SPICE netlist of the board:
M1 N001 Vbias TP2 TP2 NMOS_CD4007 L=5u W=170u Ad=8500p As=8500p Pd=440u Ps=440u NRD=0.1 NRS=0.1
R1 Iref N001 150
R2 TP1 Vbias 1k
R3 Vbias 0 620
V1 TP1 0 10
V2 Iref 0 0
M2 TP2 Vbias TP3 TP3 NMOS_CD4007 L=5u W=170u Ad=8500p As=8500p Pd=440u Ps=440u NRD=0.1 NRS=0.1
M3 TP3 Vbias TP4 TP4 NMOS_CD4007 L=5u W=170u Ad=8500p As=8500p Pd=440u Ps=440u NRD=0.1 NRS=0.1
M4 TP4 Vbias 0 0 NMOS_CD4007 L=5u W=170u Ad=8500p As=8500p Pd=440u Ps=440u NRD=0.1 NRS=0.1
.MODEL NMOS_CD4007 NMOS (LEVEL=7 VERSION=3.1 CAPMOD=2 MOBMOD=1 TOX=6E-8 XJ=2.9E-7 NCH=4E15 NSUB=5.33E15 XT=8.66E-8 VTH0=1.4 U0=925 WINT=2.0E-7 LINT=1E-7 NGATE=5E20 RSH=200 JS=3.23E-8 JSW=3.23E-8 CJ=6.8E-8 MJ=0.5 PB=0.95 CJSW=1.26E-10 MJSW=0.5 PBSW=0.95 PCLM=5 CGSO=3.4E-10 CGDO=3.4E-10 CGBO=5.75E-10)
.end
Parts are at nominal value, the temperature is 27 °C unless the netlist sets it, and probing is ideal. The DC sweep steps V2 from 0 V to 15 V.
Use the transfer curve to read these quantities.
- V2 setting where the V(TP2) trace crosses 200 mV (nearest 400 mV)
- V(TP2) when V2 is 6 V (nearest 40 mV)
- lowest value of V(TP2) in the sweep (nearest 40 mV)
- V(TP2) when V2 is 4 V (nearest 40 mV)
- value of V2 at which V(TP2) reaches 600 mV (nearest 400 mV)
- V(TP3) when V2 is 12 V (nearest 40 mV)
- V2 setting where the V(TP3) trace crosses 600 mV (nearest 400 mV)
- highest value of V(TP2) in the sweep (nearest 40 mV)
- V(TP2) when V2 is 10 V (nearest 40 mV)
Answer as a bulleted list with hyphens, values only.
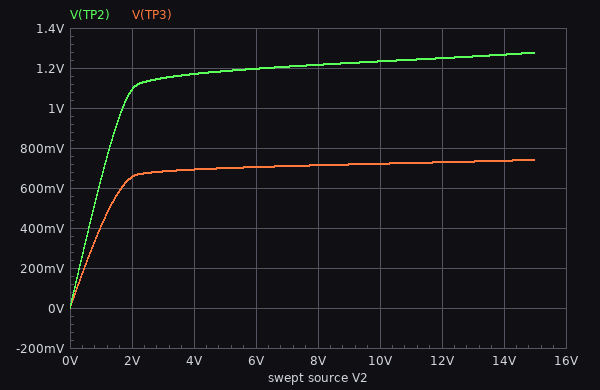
- 400 mV
- 1.20 V
- 0 V
- 1.16 V
- 800 mV
- 720 mV
- 1.6 V
- 1.28 V
- 1.24 V
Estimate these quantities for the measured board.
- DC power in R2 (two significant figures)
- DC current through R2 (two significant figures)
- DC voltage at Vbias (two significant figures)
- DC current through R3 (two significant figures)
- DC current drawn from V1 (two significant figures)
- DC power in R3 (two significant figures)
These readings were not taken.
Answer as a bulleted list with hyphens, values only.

- 38 mW
- 6.2 mA
- 3.8 V
- 6.2 mA
- 6.2 mA
- 24 mW
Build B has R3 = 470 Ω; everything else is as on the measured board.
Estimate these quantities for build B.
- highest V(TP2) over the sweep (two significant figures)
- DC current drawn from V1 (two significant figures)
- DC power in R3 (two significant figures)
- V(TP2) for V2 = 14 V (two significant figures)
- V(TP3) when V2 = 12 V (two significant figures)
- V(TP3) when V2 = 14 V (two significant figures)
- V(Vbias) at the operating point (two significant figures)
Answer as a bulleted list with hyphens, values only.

- 970 mV
- 6.8 mA
- 22 mW
- 960 mV
- 540 mV
- 550 mV
- 3.2 V
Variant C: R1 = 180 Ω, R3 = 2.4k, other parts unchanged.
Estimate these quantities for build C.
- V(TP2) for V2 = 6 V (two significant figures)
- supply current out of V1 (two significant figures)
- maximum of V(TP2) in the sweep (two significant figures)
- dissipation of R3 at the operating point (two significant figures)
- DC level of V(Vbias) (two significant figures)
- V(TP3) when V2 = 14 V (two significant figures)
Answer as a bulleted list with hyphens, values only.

- 2.7 V
- 2.9 mA
- 2.9 V
- 21 mW
- 7.1 V
- 1.7 V
